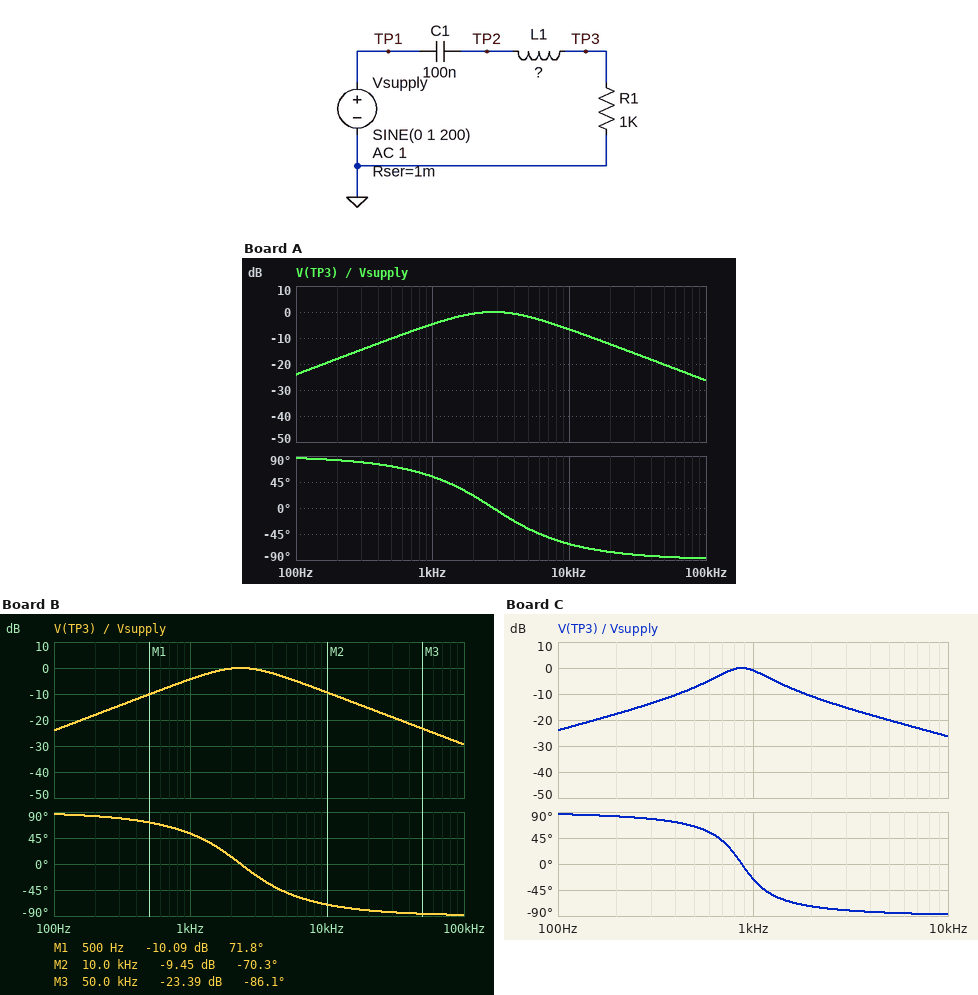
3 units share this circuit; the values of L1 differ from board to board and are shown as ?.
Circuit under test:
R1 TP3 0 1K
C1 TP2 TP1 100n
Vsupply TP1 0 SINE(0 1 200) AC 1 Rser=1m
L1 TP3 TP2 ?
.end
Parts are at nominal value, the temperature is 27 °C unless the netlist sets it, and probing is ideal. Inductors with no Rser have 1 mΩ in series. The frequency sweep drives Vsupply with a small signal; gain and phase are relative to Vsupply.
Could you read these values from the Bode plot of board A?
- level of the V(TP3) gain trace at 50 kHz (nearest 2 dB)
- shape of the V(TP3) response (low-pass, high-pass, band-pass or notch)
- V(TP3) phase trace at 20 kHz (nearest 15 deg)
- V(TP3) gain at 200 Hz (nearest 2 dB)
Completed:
-20 dB
band-pass
-75 deg
-18 dB
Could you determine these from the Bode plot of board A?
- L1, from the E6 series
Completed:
33 mH
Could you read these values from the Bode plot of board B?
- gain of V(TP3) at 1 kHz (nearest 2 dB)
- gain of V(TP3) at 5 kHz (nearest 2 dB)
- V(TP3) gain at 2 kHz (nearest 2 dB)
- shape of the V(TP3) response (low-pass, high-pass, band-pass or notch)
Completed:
-4 dB
-4 dB
0 dB
band-pass
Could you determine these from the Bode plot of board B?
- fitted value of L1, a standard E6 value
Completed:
47 mH
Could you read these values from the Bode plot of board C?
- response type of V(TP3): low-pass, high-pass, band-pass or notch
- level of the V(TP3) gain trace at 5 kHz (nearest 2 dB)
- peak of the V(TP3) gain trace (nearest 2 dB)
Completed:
band-pass
-20 dB
0 dB
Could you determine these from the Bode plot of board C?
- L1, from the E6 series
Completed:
330 mH
